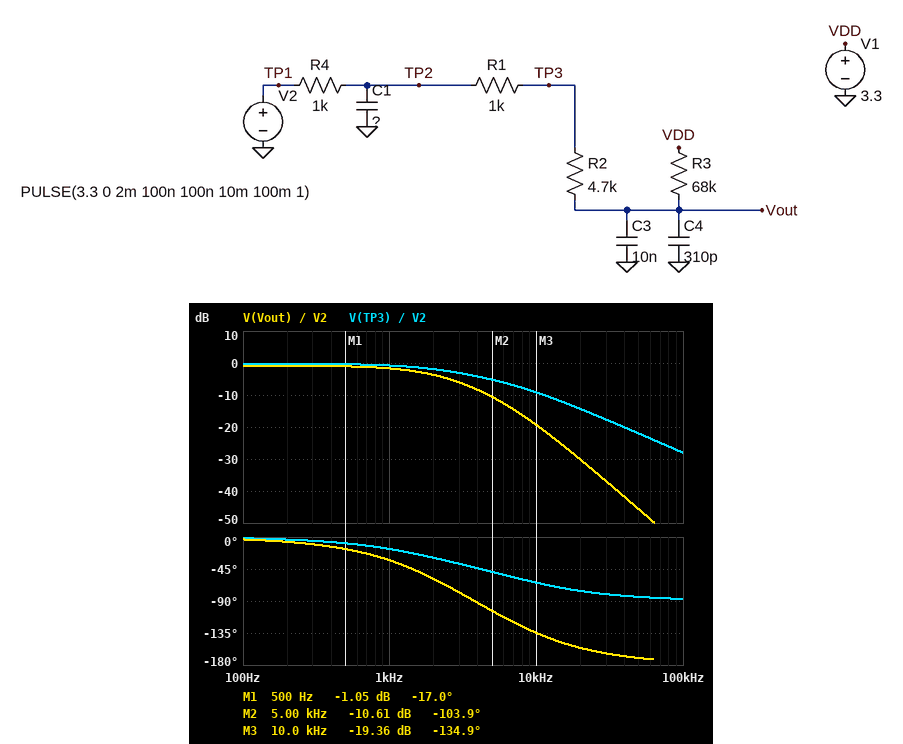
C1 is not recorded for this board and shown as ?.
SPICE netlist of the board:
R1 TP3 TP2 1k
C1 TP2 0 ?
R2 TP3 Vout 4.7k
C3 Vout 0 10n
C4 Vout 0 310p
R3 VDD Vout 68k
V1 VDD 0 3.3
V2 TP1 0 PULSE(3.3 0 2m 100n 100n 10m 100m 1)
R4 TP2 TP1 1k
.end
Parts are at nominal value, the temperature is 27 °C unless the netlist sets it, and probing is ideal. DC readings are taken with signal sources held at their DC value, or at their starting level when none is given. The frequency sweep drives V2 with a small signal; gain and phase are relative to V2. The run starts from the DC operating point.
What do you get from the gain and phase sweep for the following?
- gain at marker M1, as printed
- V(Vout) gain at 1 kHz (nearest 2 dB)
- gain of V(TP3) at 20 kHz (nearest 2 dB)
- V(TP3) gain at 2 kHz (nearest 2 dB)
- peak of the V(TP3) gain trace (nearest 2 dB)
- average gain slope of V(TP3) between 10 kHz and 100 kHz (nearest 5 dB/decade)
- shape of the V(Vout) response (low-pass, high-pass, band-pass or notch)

-1.05 dB
-2 dB
-14 dB
-2 dB
0 dB
-20 dB/decade
low-pass
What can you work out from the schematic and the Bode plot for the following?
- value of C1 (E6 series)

33 nF
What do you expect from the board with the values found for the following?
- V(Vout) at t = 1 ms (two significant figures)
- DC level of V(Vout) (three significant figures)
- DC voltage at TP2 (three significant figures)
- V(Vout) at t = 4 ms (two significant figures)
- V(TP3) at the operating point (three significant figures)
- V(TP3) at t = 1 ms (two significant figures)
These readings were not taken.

3.3 V
3.30 V
3.30 V
300 mV
3.30 V
3.3 V
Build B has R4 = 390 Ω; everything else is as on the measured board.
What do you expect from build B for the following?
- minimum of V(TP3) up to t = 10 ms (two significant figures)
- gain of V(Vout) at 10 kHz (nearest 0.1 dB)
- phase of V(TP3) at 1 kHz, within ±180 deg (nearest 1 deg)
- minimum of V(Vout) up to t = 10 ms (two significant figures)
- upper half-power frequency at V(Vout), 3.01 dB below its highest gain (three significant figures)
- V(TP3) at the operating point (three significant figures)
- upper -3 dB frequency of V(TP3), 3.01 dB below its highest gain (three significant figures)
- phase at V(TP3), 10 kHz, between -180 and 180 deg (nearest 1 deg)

62 mV
-14.3 dB
-9 deg
270 mV
2.62 kHz
3.30 V
7.30 kHz
-41 deg
